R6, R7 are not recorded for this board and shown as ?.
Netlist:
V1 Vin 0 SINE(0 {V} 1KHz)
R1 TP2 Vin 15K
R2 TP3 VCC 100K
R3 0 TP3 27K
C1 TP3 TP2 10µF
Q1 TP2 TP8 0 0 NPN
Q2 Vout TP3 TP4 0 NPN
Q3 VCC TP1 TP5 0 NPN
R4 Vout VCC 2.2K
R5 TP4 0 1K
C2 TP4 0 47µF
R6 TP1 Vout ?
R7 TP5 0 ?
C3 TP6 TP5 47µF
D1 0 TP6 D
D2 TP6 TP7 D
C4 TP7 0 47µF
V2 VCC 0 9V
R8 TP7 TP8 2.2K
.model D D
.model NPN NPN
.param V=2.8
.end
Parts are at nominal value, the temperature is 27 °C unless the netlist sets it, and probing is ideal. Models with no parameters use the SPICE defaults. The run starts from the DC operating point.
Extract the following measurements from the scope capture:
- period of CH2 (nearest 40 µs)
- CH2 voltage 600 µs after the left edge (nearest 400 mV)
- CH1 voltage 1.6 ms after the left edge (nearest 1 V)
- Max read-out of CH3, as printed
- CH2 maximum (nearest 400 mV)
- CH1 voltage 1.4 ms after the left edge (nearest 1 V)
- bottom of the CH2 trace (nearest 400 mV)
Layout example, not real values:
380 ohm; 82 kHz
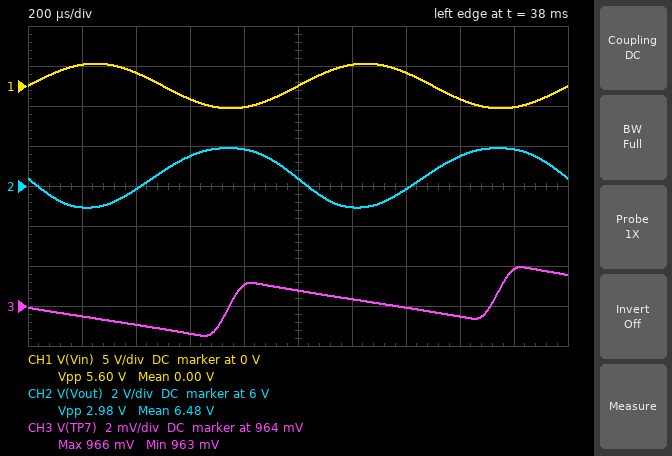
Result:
1.00 ms; 7.6 V; -2 V; 966 mV; 8.0 V; 2 V; 4.8 V
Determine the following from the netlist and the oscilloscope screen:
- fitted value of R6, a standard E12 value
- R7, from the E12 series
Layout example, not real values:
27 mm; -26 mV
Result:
4.7 kΩ; 220 Ω
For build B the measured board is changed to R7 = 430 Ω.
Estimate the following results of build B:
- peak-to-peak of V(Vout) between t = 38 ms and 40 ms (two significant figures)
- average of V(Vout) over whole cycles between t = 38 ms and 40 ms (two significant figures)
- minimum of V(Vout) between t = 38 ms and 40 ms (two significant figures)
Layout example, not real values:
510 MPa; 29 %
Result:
2.8 V; 6.7 V; 5.2 V
